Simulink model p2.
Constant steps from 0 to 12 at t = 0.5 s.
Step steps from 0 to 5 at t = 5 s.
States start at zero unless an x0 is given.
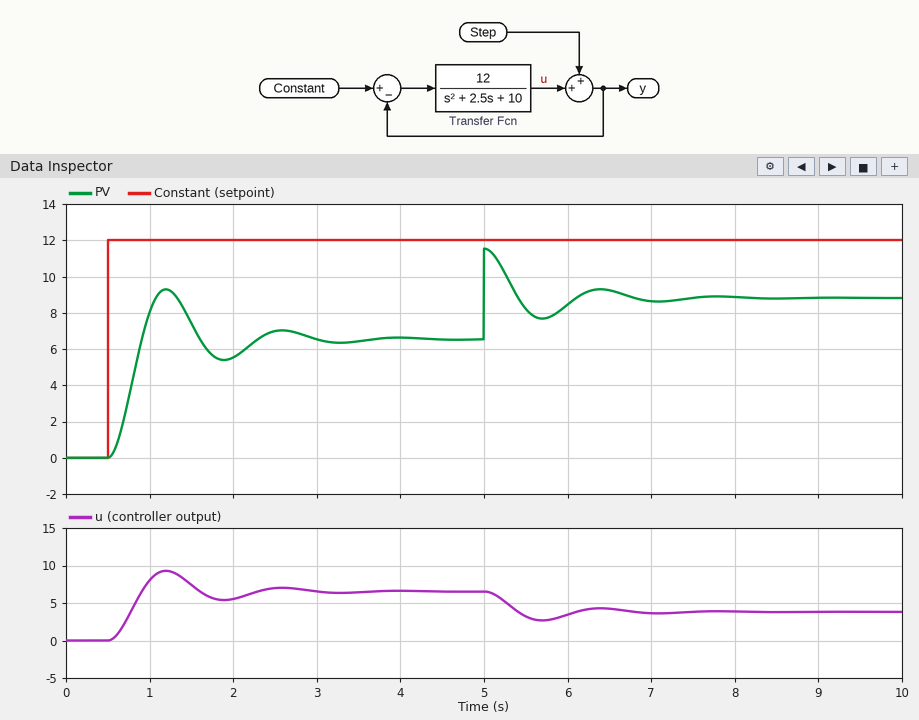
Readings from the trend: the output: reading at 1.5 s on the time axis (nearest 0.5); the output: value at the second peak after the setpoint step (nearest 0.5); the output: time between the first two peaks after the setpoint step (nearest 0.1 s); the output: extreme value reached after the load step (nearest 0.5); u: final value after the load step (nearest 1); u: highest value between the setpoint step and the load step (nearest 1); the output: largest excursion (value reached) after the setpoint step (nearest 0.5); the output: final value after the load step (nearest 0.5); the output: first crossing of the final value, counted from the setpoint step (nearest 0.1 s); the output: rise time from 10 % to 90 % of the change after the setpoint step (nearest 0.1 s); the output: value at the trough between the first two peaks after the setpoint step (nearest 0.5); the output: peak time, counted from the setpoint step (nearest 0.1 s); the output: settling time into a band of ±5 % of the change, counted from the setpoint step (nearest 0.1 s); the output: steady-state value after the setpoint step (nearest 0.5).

7.5
7.0
1.4 s
11.5
4
9
9.5
9.0
0.4 s
0.3 s
5.5
0.7 s
2.3 s
6.5
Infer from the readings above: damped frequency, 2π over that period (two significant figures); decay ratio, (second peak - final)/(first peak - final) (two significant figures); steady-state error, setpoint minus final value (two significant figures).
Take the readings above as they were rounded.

4.5 rad/s
0.17
5.5
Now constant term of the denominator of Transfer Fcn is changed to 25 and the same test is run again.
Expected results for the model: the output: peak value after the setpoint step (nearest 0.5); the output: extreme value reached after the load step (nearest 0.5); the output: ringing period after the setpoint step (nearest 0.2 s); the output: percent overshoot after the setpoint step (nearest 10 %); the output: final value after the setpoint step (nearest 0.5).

6.0
9.0
1.0 s
50 %
4.0
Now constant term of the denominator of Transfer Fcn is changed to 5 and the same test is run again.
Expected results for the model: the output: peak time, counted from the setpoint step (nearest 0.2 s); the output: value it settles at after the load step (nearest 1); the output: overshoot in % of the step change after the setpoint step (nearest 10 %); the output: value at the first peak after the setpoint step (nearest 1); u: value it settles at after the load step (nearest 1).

0.8 s
10
40 %
12
5
